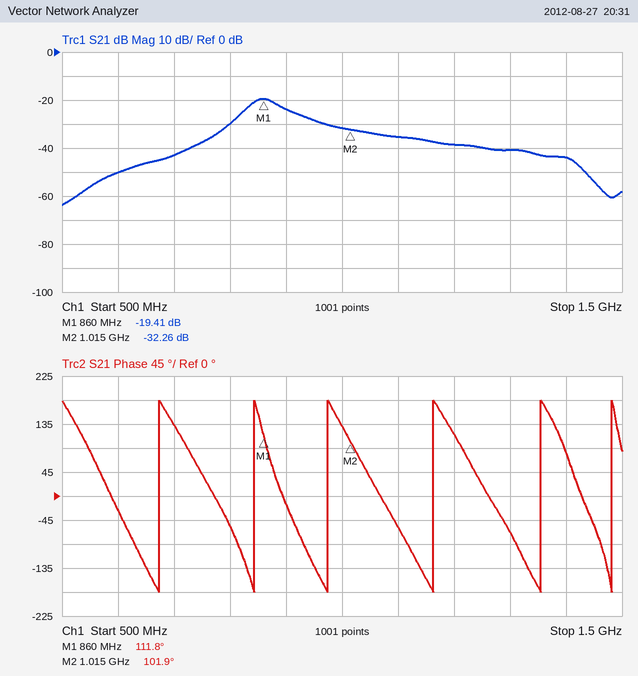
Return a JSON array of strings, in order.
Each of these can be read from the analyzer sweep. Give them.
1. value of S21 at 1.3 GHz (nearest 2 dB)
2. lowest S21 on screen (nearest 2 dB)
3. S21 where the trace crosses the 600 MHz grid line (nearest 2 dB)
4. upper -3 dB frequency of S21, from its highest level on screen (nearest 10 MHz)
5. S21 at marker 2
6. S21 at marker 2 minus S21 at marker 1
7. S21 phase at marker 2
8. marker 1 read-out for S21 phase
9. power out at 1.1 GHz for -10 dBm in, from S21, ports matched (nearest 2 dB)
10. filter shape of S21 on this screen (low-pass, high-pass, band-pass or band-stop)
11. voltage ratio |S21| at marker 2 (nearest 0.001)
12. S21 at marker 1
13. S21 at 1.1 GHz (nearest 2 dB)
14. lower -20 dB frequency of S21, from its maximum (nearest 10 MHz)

["-40 dB", "-64 dB", "-50 dB", "890 MHz", "-32.26 dB", "-12.85 dB", "101.9°", "111.8°", "-46 dBm", "band-pass", "0.024", "-19.41 dB", "-36 dB", "730 MHz"]
